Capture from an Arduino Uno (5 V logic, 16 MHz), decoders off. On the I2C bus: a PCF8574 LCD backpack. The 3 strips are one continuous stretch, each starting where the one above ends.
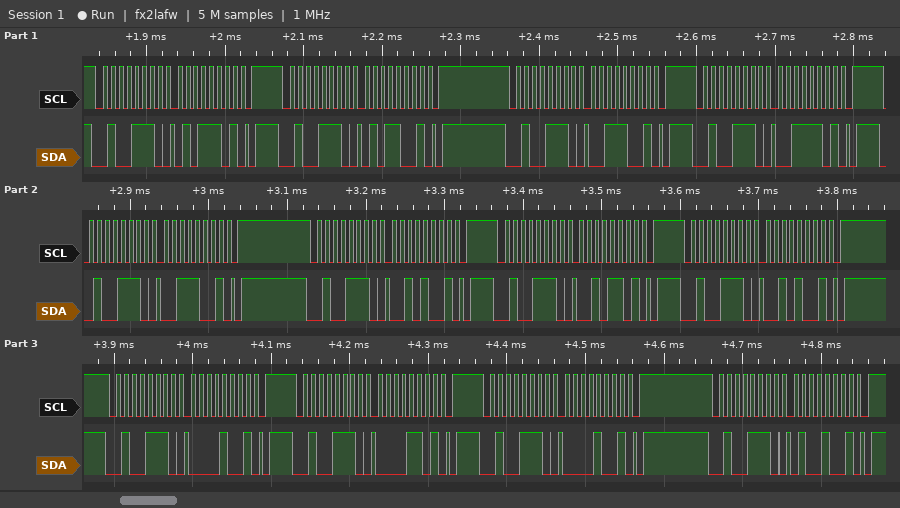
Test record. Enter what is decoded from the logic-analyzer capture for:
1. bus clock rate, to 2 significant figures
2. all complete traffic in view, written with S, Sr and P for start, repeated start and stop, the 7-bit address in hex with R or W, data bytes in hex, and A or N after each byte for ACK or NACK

100 kHz
S 27W A 5D A P S 27W A 59 A P S 27W A 39 A P S 27W A 3D A P S 27W A 39 A P S 27W A 29 A P S 27W A 2D A P S 27W A 29 A P S 27W A 09 A P S 27W A 0D A P S 27W A 09 A P S 27W A 49 A P
